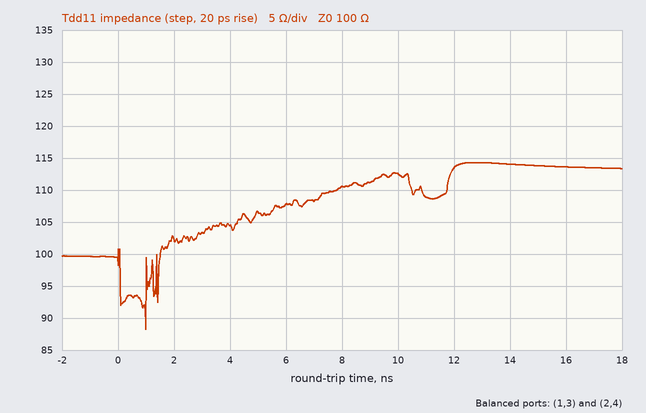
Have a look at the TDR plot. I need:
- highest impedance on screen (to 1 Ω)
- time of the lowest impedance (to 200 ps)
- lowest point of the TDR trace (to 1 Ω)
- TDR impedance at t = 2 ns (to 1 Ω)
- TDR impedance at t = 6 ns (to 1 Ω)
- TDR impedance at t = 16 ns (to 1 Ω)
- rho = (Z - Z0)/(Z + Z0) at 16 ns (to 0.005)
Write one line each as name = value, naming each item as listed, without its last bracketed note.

highest impedance on screen = 114 Ω
time of the lowest impedance = 1.0 ns
lowest point of the TDR trace = 88 Ω
TDR impedance at t = 2 ns = 102 Ω
TDR impedance at t = 6 ns = 108 Ω
TDR impedance at t = 16 ns = 114 Ω
rho = (Z - Z0)/(Z + Z0) at 16 ns = +0.065
